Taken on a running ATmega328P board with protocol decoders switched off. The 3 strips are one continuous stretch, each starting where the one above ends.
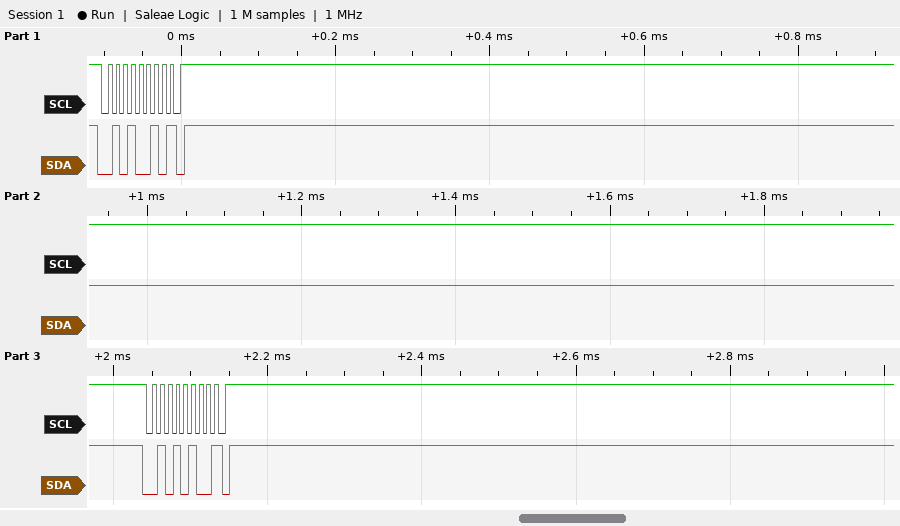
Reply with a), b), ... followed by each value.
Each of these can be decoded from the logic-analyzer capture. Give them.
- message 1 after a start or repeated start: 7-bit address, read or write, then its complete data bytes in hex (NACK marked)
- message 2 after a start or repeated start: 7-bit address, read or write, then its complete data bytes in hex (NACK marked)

a) 0x29 write NACK
b) 0x2A write NACK
